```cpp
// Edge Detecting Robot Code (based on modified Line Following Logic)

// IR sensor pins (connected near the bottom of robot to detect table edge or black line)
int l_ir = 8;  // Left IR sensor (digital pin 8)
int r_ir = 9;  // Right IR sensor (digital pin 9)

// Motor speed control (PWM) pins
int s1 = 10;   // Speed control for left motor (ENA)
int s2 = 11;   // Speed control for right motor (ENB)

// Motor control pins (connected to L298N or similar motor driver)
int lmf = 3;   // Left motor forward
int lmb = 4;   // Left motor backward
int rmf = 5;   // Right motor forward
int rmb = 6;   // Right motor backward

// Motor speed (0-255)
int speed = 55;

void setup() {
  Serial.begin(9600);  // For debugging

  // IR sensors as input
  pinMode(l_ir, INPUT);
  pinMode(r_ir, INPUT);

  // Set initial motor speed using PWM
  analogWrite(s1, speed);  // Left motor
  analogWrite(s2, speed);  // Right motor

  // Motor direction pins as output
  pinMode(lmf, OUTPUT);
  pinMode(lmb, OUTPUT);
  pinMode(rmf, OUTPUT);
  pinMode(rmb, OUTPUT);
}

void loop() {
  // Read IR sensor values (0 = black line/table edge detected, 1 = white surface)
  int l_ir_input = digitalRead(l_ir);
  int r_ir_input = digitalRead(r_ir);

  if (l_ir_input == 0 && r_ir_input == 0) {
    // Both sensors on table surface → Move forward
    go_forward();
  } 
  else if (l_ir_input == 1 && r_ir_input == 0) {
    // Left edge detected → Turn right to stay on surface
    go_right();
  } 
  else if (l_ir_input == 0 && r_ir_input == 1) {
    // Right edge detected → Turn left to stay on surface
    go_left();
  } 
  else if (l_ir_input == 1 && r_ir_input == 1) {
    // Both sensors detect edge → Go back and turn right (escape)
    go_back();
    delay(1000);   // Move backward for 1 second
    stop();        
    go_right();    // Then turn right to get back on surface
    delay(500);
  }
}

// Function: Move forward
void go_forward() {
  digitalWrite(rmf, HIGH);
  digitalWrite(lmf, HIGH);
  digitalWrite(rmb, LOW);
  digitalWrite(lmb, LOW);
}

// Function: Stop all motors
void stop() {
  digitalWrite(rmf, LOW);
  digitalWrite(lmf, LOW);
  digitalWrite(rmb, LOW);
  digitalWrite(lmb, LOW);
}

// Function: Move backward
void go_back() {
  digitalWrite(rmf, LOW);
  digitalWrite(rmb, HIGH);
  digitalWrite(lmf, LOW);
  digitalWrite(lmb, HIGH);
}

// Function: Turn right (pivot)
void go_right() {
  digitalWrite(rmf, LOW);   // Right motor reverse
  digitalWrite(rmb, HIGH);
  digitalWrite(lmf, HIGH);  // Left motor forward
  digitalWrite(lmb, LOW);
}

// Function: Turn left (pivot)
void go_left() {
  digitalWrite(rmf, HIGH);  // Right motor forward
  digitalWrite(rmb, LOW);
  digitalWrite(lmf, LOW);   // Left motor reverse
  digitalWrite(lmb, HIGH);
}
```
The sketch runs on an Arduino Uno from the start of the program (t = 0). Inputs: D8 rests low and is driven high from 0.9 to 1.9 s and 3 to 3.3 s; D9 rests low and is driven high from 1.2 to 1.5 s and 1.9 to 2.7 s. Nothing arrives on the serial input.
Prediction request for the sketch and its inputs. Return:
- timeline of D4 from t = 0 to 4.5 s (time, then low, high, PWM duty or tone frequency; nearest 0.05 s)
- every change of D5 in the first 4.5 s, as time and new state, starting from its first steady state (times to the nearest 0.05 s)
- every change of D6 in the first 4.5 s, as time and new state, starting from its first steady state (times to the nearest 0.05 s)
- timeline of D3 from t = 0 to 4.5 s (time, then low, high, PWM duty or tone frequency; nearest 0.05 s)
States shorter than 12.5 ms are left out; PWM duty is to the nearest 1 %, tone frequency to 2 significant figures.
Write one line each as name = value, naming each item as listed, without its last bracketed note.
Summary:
timeline of D4 from t = 0 to 4.5 s = 0 s low; 1.2 s high; 2.2 s low
every change of D5 in the first 4.5 s, as time and new state, starting from its first steady state = 0 s high; 0.9 s low; 2.7 s high; 3 s low; 3.3 s high
every change of D6 in the first 4.5 s, as time and new state, starting from its first steady state = 0 s low; 0.9 s high; 2.7 s low; 3 s high; 3.3 s low
timeline of D3 from t = 0 to 4.5 s = 0 s high; 1.2 s low; 2.2 s high
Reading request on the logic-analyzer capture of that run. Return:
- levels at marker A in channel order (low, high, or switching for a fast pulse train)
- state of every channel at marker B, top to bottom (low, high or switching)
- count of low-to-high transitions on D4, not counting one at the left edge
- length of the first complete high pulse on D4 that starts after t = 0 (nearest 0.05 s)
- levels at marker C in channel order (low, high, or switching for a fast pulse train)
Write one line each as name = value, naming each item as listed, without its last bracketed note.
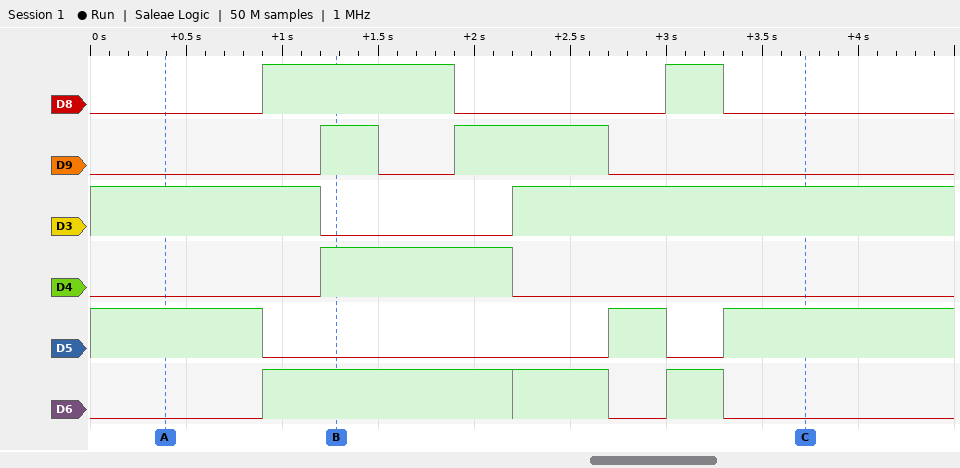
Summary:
levels at marker A in channel order = D8 low, D9 low, D3 high, D4 low, D5 high, D6 low
state of every channel at marker B, top to bottom = D8 high, D9 high, D3 low, D4 high, D5 low, D6 high
count of low-to-high transitions on D4, not counting one at the left edge = 1
length of the first complete high pulse on D4 that starts after t = 0 = 1.00 s
levels at marker C in channel order = D8 low, D9 low, D3 high, D4 low, D5 high, D6 low
